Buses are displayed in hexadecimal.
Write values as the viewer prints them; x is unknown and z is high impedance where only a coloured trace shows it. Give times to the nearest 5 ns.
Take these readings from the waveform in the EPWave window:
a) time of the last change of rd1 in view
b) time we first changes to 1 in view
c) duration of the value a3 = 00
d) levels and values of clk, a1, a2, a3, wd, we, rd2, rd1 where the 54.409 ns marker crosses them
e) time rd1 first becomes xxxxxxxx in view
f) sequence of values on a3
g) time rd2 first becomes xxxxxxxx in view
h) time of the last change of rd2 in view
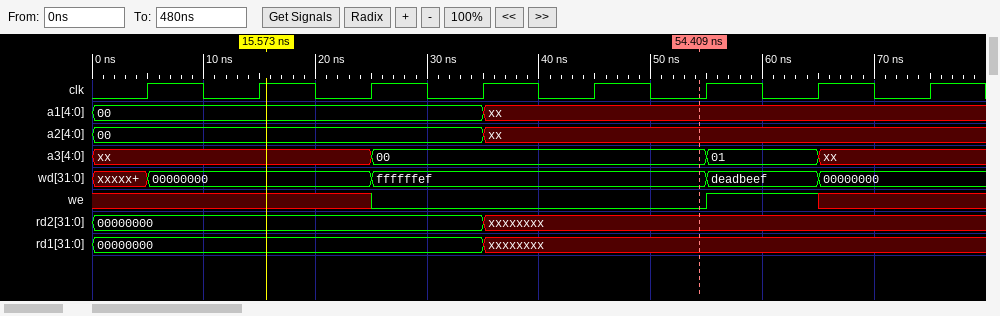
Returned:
35 ns
55 ns
30 ns
clk=0, a1=xx, a2=xx, a3=00, wd=ffffffef, we=0, rd2=xxxxxxxx, rd1=xxxxxxxx
35 ns
xx, 00, 01, xx
35 ns
35 ns
